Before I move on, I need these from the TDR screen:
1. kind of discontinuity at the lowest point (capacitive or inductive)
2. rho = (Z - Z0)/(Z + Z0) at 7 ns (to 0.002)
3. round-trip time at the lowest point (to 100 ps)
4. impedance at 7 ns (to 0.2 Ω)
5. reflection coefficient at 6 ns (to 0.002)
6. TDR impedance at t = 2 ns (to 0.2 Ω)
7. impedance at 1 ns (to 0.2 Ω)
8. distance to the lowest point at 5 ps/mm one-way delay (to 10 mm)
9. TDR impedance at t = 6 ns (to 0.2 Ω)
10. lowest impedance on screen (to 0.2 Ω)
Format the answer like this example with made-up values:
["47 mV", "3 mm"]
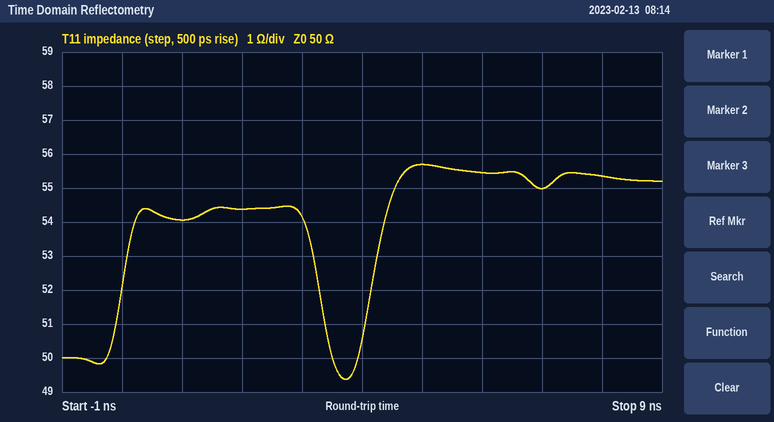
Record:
["capacitive", "+0.048", "3.7 ns", "55.0 Ω", "+0.052", "54.4 Ω", "54.0 Ω", "370 mm", "55.4 Ω", "49.4 Ω"]
